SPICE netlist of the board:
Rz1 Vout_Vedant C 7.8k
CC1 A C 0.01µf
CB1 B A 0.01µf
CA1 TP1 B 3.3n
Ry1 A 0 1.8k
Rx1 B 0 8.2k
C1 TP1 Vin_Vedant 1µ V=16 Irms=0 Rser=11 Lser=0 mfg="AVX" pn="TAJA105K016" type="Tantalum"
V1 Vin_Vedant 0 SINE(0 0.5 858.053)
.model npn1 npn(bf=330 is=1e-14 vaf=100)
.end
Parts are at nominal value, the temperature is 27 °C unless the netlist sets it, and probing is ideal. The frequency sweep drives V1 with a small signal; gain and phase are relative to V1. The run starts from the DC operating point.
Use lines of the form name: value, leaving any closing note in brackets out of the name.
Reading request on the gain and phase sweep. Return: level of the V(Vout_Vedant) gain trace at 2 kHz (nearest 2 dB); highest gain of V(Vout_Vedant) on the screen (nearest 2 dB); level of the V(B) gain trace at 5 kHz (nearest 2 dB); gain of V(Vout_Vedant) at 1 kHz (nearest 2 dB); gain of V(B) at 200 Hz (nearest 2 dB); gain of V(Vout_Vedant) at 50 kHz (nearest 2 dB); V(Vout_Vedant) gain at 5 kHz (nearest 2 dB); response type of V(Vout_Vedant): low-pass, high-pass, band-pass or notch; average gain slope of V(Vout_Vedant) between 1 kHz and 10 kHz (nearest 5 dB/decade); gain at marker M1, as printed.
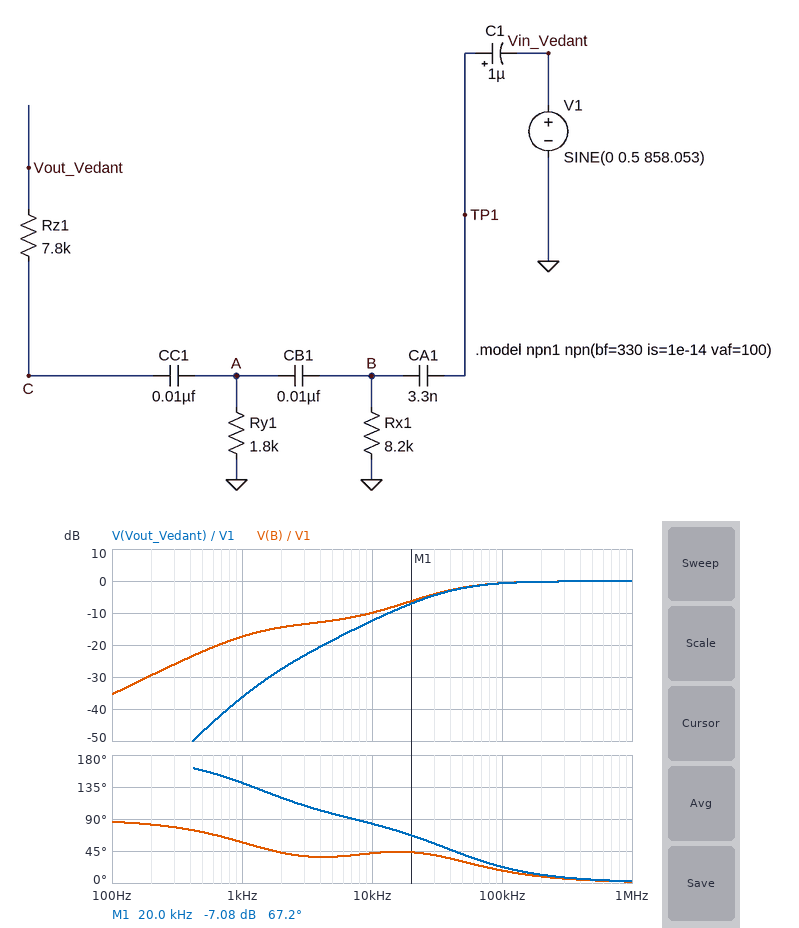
level of the V(Vout_Vedant) gain trace at 2 kHz: -28 dB
highest gain of V(Vout_Vedant) on the screen: 0 dB
level of the V(B) gain trace at 5 kHz: -12 dB
gain of V(Vout_Vedant) at 1 kHz: -36 dB
gain of V(B) at 200 Hz: -30 dB
gain of V(Vout_Vedant) at 50 kHz: -2 dB
V(Vout_Vedant) gain at 5 kHz: -18 dB
response type of V(Vout_Vedant): low-pass, high-pass, band-pass or notch: high-pass
average gain slope of V(Vout_Vedant) between 1 kHz and 10 kHz: 25 dB/decade
gain at marker M1, as printed: -7.08 dB
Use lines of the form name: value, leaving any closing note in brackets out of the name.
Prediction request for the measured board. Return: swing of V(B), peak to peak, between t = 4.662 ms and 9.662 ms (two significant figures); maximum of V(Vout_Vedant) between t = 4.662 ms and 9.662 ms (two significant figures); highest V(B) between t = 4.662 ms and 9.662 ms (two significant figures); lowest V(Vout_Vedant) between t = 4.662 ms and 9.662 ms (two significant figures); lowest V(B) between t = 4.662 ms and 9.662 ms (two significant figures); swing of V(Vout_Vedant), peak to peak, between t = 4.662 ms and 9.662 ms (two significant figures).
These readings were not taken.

swing of V(B), peak to peak, between t = 4.662 ms and 9.662 ms: 120 mV
maximum of V(Vout_Vedant) between t = 4.662 ms and 9.662 ms: 5.9 mV
highest V(B) between t = 4.662 ms and 9.662 ms: 61 mV
lowest V(Vout_Vedant) between t = 4.662 ms and 9.662 ms: -5.9 mV
lowest V(B) between t = 4.662 ms and 9.662 ms: -61 mV
swing of V(Vout_Vedant), peak to peak, between t = 4.662 ms and 9.662 ms: 12 mV
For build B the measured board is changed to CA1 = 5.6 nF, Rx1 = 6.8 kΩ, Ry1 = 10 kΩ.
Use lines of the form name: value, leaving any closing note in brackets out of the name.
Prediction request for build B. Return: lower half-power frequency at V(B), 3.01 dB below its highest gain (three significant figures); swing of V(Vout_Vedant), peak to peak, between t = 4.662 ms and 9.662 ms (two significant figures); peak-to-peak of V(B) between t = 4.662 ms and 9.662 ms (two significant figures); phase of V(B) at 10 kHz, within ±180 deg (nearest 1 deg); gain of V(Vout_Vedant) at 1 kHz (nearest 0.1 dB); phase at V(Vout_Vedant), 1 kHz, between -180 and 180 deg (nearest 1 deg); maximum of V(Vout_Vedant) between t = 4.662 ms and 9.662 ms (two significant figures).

lower half-power frequency at V(B), 3.01 dB below its highest gain: 7.54 kHz
swing of V(Vout_Vedant), peak to peak, between t = 4.662 ms and 9.662 ms: 77 mV
peak-to-peak of V(B) between t = 4.662 ms and 9.662 ms: 160 mV
phase of V(B) at 10 kHz, within ±180 deg: 34 deg
gain of V(Vout_Vedant) at 1 kHz: -20.3 dB
phase at V(Vout_Vedant), 1 kHz, between -180 and 180 deg: 123 deg
maximum of V(Vout_Vedant) between t = 4.662 ms and 9.662 ms: 39 mV
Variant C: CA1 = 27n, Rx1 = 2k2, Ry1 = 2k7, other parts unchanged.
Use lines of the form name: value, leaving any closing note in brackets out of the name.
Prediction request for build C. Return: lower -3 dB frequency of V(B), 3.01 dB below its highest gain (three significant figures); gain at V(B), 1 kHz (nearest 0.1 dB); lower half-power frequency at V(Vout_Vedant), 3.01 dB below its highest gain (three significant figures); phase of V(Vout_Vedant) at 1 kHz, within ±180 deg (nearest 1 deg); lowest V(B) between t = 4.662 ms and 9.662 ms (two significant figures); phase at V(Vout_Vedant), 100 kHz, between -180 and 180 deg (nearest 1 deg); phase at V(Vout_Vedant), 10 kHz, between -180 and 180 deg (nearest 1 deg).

lower -3 dB frequency of V(B), 3.01 dB below its highest gain: 5.05 kHz
gain at V(B), 1 kHz: -9.9 dB
lower half-power frequency at V(Vout_Vedant), 3.01 dB below its highest gain: 9.37 kHz
phase of V(Vout_Vedant) at 1 kHz, within ±180 deg: 144 deg
lowest V(B) between t = 4.662 ms and 9.662 ms: -140 mV
phase at V(Vout_Vedant), 100 kHz, between -180 and 180 deg: 6 deg
phase at V(Vout_Vedant), 10 kHz, between -180 and 180 deg: 52 deg
